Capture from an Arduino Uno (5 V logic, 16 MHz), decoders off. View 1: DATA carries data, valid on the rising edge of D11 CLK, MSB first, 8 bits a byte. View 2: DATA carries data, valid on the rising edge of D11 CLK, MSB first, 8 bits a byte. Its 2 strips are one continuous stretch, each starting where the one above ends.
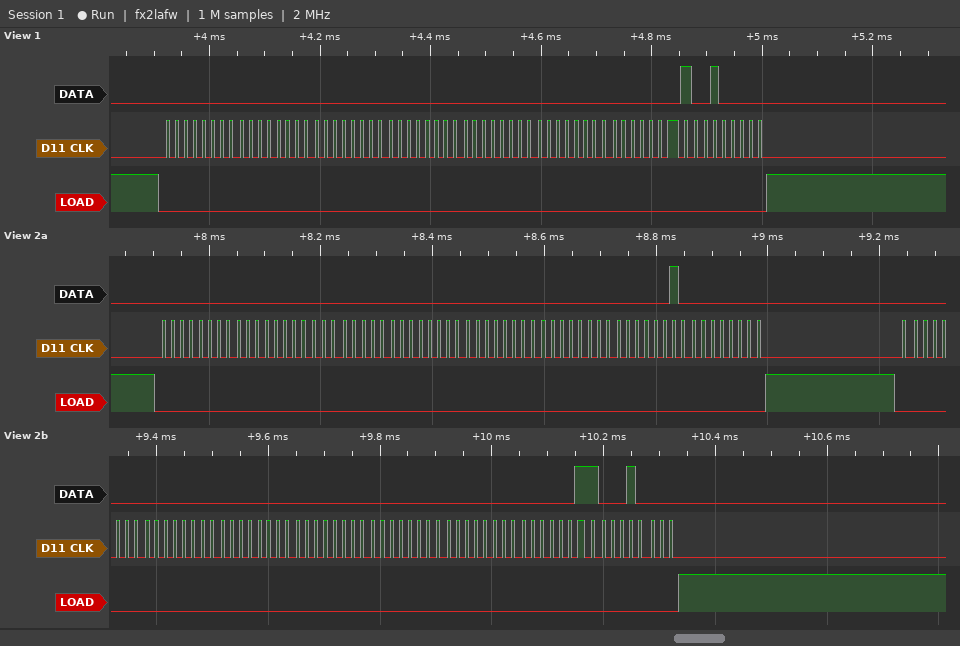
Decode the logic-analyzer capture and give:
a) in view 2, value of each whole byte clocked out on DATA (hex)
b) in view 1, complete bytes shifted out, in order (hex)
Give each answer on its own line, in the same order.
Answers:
00 00 00 00 00 00 02 00 00 00 00 00 00 00 03 10
00 00 00 00 00 00 01 20
